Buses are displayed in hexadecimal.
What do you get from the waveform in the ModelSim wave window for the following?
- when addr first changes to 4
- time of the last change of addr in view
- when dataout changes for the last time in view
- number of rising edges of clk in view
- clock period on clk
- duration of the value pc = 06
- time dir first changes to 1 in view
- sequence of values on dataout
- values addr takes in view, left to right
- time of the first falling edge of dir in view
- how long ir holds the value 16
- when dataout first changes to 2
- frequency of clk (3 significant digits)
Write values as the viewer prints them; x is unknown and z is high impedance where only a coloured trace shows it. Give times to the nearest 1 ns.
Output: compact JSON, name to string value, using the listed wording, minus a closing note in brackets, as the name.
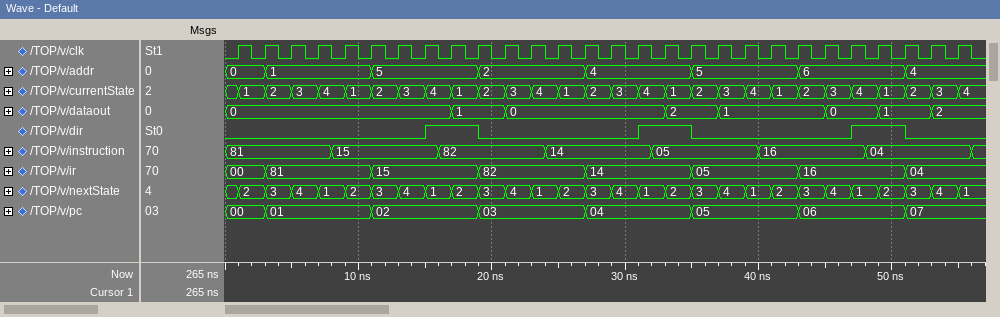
{"when addr first changes to 4": "27 ns", "time of the last change of addr in view": "51 ns", "when dataout changes for the last time in view": "53 ns", "number of rising edges of clk in view": "28", "clock period on clk": "2 ns", "duration of the value pc = 06": "8 ns", "time dir first changes to 1 in view": "15 ns", "sequence of values on dataout": "0, 1, 0, 2, 1, 0, 1, 2", "values addr takes in view, left to right": "0, 1, 5, 2, 4, 5, 6, 4", "time of the first falling edge of dir in view": "19 ns", "how long ir holds the value 16": "8 ns", "when dataout first changes to 2": "33 ns", "frequency of clk": "500 MHz"}
